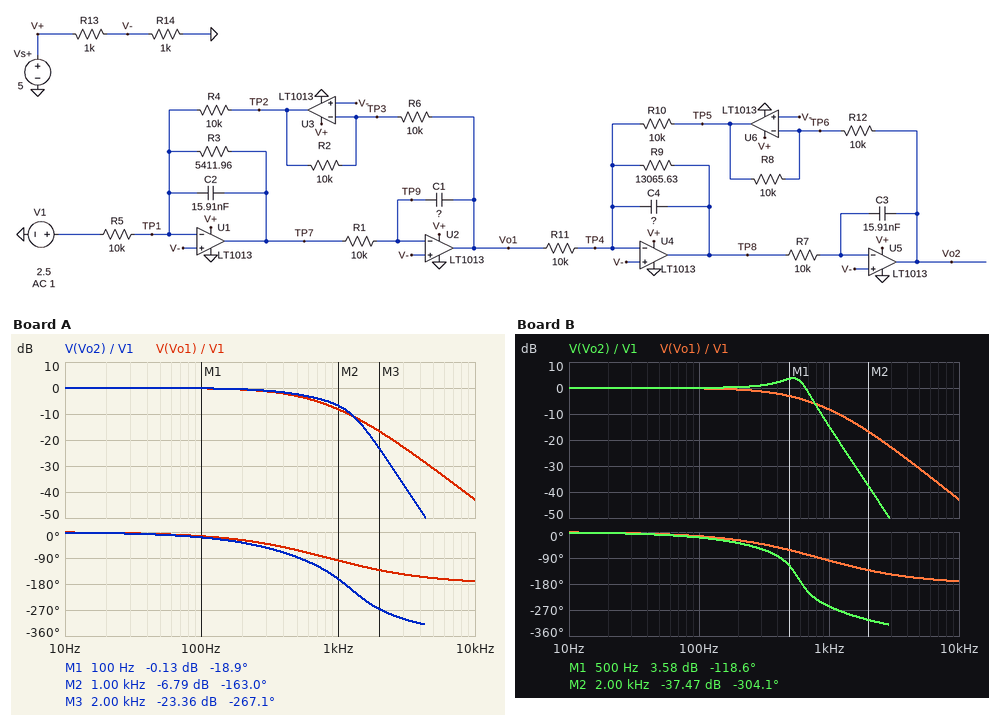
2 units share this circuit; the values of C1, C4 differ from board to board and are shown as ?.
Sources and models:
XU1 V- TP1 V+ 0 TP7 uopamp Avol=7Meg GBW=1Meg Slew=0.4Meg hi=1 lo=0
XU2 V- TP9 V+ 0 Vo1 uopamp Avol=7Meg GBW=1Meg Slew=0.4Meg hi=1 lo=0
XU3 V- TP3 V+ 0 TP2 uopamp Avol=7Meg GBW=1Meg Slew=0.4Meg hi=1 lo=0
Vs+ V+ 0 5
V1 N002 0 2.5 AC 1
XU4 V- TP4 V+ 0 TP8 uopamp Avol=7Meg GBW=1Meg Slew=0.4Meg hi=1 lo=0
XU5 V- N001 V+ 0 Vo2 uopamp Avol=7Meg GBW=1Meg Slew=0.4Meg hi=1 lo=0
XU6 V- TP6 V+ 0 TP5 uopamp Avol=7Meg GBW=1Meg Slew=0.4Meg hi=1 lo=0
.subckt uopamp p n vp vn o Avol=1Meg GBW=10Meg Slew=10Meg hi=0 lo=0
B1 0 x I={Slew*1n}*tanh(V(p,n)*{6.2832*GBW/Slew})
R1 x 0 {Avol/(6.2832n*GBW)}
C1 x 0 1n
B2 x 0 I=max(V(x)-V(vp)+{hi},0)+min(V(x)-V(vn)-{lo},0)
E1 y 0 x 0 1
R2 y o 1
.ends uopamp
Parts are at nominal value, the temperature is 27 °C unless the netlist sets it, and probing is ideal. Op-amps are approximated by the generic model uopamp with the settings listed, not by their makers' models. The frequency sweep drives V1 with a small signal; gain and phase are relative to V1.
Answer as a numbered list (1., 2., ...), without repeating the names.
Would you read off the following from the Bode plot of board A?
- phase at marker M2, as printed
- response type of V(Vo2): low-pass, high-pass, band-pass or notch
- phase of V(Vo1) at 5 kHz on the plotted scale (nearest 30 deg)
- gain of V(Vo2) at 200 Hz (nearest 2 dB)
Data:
1. -163.0 deg
2. low-pass
3. -150 deg
4. 0 dB
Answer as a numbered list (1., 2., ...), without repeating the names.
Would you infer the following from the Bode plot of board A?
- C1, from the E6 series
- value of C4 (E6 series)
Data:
1. 22 nF
2. 10 nF
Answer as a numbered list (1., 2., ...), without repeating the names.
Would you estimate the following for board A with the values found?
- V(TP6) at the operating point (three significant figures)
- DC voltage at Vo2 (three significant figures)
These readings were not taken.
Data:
1. 2.50 V
2. 2.50 V
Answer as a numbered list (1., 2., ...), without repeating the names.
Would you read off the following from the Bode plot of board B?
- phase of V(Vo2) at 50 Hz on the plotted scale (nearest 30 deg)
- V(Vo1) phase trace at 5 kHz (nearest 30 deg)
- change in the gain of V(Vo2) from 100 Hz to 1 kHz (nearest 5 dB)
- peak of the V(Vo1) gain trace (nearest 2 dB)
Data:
1. 0 deg
2. -150 deg
3. -15 dB
4. 0 dB
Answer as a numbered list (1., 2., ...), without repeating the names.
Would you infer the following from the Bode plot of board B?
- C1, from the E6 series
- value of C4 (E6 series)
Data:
1. 22 nF
2. 47 nF
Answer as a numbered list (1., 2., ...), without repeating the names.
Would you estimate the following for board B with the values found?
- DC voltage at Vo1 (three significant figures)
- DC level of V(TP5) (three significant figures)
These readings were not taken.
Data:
1. 2.50 V
2. 2.50 V
